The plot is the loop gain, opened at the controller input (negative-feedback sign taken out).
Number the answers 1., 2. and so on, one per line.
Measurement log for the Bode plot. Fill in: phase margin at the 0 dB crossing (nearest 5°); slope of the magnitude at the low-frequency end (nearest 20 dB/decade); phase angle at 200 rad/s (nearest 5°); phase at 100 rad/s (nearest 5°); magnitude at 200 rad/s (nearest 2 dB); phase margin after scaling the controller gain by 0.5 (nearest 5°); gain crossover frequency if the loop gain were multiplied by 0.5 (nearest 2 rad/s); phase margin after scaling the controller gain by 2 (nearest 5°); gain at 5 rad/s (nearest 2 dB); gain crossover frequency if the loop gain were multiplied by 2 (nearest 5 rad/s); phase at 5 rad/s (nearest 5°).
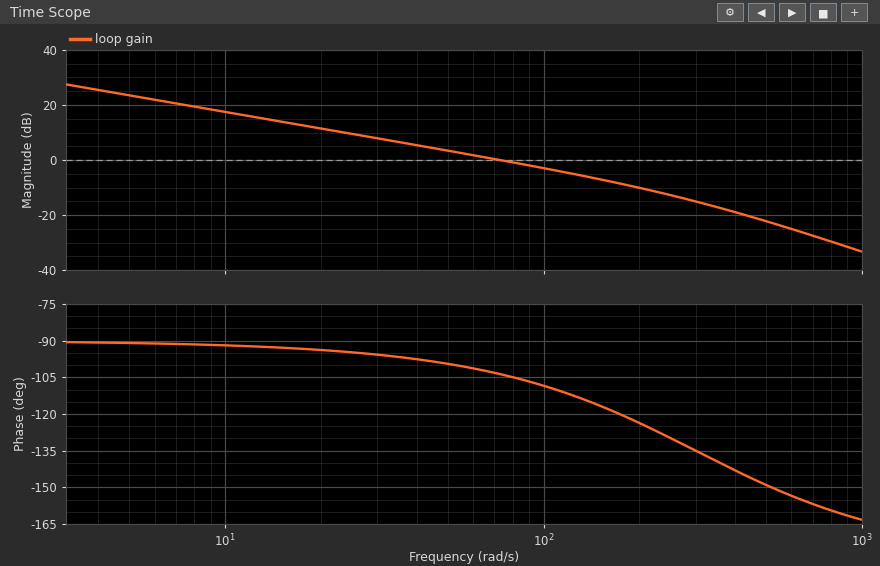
1. 75°
2. -20 dB/decade
3. -125°
4. -110°
5. -10 dB
6. 85°
7. 38 rad/s
8. 65°
9. 24 dB
10. 135 rad/s
11. -90°
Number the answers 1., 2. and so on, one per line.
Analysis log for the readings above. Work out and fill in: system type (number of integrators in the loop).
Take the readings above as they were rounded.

1. 1
